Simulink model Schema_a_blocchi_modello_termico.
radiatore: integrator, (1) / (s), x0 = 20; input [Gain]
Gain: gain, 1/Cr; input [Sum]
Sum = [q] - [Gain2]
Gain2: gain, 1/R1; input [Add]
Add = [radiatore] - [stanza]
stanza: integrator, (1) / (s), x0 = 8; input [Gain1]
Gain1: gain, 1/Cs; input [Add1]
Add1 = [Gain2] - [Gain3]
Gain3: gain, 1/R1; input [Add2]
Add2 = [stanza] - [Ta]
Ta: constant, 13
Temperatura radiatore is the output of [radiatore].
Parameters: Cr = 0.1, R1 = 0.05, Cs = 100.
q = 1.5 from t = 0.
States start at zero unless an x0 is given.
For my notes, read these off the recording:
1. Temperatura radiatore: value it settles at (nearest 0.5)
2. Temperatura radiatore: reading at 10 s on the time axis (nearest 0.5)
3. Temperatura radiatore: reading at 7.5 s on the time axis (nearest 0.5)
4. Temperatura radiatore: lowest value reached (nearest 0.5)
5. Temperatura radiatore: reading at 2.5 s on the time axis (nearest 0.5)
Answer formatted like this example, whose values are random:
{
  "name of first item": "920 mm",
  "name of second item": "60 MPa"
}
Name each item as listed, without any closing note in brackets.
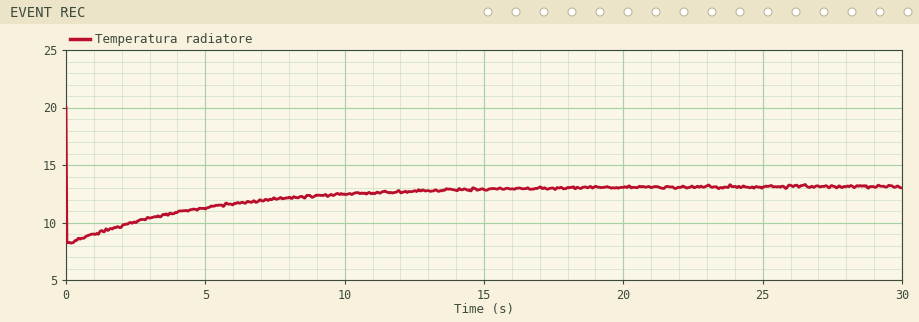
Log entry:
{
  "Temperatura radiatore: value it settles at": "13.0",
  "Temperatura radiatore: reading at 10 s on the time axis": "12.5",
  "Temperatura radiatore: reading at 7.5 s on the time axis": "12.0",
  "Temperatura radiatore: lowest value reached": "8.0",
  "Temperatura radiatore: reading at 2.5 s on the time axis": "10.0"
}
